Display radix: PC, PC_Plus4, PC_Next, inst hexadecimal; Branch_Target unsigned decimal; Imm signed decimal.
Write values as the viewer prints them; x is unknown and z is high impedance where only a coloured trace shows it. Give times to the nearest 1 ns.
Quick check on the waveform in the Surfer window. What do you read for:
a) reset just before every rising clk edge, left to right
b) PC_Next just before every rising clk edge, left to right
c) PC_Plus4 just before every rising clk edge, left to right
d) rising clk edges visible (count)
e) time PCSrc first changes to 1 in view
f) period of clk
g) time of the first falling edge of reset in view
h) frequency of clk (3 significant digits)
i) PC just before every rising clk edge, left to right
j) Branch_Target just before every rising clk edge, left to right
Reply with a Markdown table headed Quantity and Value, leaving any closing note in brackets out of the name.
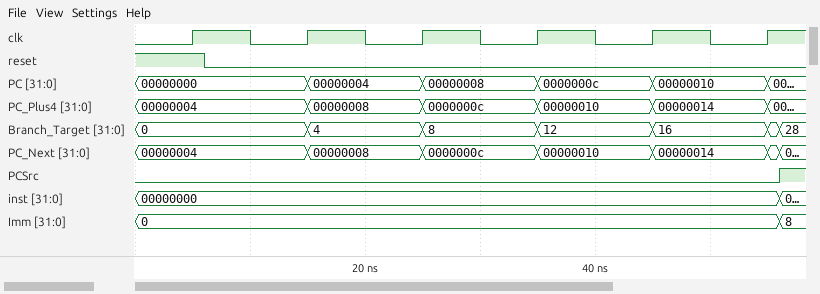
| Quantity | Value |
|---|---|
| reset just before every rising clk edge, left to right | 1 0 0 0 0 0 |
| PC_Next just before every rising clk edge, left to right | 00000004, 00000004, 00000008, 0000000c, 00000010, 00000014 |
| PC_Plus4 just before every rising clk edge, left to right | 00000004, 00000004, 00000008, 0000000c, 00000010, 00000014 |
| rising clk edges visible | 6 |
| time PCSrc first changes to 1 in view | 56 ns |
| period of clk | 10 ns |
| time of the first falling edge of reset in view | 6 ns |
| frequency of clk | 100 MHz |
| PC just before every rising clk edge, left to right | 00000000, 00000000, 00000004, 00000008, 0000000c, 00000010 |
| Branch_Target just before every rising clk edge, left to right | 0, 0, 4, 8, 12, 16 |
